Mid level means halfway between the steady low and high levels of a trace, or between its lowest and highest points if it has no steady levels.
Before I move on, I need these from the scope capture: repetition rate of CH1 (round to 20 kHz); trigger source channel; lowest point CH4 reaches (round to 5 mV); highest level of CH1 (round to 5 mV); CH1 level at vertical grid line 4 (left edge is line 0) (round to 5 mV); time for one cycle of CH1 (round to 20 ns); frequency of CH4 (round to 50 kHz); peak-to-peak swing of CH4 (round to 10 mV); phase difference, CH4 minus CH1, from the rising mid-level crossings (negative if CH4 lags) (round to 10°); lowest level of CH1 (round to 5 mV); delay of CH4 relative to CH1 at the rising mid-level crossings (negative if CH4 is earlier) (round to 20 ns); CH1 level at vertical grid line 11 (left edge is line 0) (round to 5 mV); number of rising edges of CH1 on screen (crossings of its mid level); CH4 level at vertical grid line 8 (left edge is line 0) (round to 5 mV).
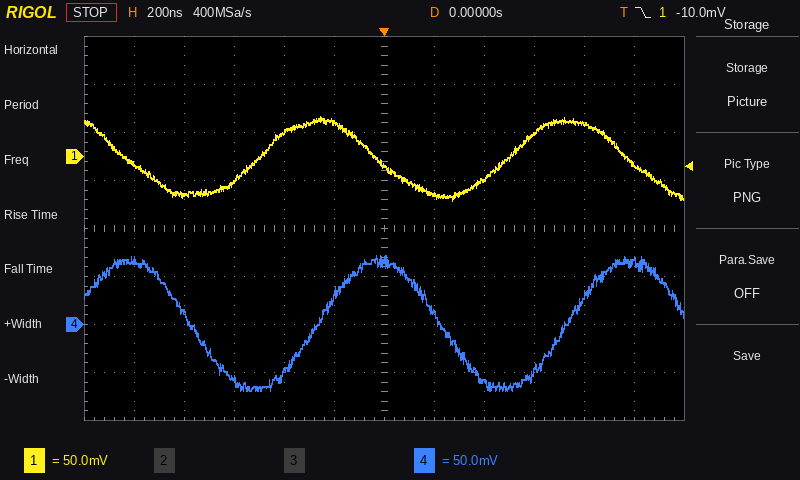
1.00 MHz
CH1
-70 mV
40 mV
25 mV
1.00 µs
1.00 MHz
140 mV
-90°
-45 mV
+240 ns
-10 mV
2
-60 mV
